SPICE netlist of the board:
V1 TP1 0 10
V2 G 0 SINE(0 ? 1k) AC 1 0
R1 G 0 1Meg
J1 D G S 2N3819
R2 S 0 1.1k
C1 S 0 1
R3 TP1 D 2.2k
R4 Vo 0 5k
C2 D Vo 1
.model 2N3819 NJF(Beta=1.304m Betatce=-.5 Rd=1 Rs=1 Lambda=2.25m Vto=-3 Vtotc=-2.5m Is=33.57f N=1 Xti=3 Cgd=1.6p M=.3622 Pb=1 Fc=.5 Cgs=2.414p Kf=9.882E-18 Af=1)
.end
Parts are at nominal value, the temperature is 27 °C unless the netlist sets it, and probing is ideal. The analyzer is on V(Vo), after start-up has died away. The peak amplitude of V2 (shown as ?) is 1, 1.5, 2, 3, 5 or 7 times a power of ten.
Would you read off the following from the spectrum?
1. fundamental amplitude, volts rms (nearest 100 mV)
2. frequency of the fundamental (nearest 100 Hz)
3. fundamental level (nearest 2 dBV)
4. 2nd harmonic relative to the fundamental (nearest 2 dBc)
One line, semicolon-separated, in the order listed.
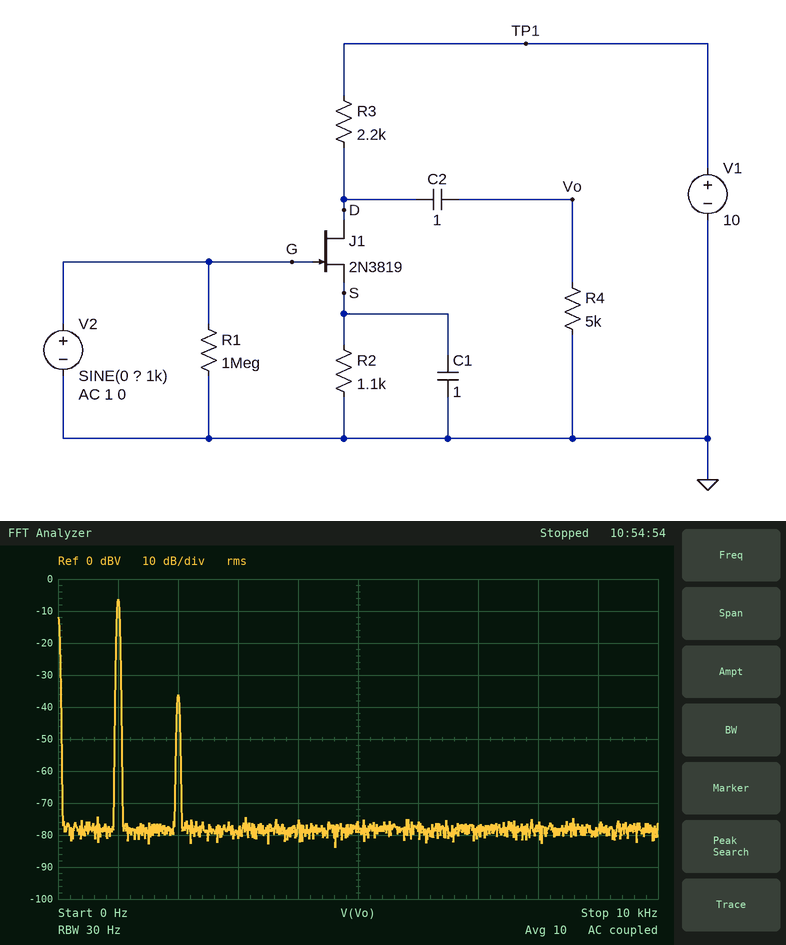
500 mV; 1.0 kHz; -6 dBV; -30 dBc
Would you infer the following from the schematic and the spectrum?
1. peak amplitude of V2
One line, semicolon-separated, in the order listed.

150 mV
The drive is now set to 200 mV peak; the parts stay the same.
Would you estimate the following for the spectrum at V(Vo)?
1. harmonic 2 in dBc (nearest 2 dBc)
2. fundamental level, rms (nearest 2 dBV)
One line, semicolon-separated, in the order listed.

-28 dBc; -4 dBV
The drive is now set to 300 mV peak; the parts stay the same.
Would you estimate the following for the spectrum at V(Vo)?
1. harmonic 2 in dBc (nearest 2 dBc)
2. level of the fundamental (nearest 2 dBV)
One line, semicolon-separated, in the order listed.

-24 dBc; 0 dBV
